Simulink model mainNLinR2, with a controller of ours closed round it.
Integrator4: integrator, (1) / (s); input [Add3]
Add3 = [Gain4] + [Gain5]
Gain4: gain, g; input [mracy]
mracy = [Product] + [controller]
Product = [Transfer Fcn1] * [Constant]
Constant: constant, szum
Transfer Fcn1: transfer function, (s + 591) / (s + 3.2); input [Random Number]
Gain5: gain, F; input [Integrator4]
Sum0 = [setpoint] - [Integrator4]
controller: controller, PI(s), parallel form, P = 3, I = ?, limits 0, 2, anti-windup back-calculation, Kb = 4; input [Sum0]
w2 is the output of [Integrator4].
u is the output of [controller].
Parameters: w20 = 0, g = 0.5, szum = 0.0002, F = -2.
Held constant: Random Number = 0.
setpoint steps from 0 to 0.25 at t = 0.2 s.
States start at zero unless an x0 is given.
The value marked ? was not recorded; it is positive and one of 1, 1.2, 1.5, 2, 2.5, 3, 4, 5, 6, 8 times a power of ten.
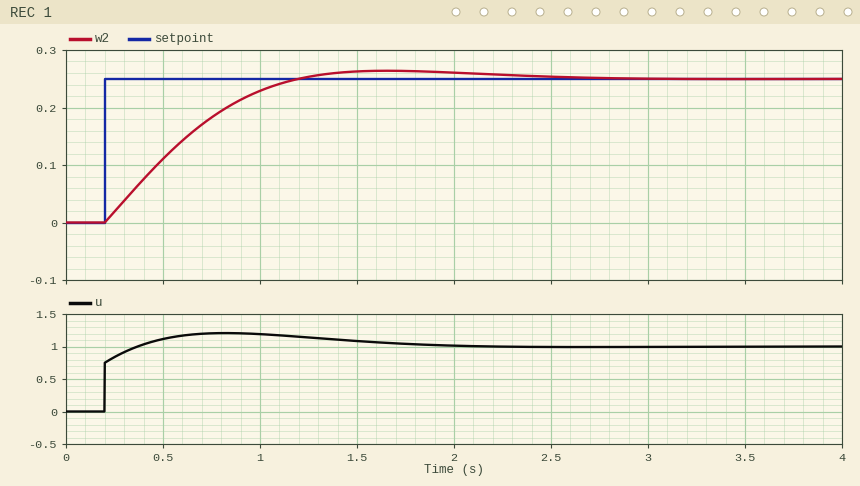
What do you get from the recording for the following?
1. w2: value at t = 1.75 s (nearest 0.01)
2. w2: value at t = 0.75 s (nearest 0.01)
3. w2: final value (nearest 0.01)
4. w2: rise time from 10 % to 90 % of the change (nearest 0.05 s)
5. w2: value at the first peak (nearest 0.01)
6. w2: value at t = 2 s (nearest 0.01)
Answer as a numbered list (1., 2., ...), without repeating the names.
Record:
1. 0.26
2. 0.18
3. 0.25
4. 0.70 s
5. 0.26
6. 0.26
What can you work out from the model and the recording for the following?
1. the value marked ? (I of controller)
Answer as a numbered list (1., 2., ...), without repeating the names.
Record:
1. 12
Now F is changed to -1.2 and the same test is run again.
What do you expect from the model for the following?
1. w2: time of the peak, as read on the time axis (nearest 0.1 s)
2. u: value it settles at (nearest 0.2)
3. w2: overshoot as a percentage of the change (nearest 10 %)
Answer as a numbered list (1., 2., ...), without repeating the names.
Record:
1. 1.4 s
2. 0.6
3. 20 %
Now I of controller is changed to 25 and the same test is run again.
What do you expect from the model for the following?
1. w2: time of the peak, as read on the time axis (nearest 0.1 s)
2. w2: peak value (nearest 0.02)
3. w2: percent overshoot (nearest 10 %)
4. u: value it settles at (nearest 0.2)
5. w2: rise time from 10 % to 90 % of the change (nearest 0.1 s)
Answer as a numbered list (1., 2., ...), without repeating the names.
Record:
1. 1.1 s
2. 0.30
3. 20 %
4. 1.0
5. 0.4 s
